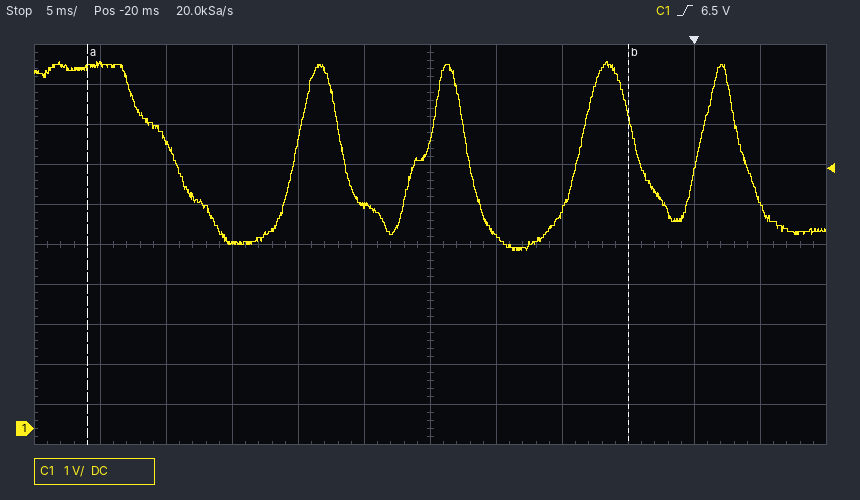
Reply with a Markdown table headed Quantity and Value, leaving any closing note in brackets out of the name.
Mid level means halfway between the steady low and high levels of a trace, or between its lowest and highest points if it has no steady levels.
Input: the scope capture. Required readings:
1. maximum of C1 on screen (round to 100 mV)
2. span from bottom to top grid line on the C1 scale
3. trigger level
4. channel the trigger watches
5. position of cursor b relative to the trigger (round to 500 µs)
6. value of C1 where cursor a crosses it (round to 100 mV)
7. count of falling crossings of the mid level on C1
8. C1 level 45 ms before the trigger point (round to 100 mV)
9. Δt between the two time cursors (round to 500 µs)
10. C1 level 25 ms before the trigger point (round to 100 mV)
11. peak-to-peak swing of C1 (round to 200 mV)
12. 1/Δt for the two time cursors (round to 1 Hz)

| Quantity | Value |
|---|---|
| maximum of C1 on screen | 9.2 V |
| span from bottom to top grid line on the C1 scale | 10 V |
| trigger level | 6.5 V |
| channel the trigger watches | C1 |
| position of cursor b relative to the trigger | -5.0 ms |
| value of C1 where cursor a crosses it | 9.0 V |
| count of falling crossings of the mid level on C1 | 5 |
| C1 level 45 ms before the trigger point | 9.1 V |
| Δt between the two time cursors | 41.0 ms |
| C1 level 25 ms before the trigger point | 5.6 V |
| peak-to-peak swing of C1 | 4.8 V |
| 1/Δt for the two time cursors | 24 Hz |
